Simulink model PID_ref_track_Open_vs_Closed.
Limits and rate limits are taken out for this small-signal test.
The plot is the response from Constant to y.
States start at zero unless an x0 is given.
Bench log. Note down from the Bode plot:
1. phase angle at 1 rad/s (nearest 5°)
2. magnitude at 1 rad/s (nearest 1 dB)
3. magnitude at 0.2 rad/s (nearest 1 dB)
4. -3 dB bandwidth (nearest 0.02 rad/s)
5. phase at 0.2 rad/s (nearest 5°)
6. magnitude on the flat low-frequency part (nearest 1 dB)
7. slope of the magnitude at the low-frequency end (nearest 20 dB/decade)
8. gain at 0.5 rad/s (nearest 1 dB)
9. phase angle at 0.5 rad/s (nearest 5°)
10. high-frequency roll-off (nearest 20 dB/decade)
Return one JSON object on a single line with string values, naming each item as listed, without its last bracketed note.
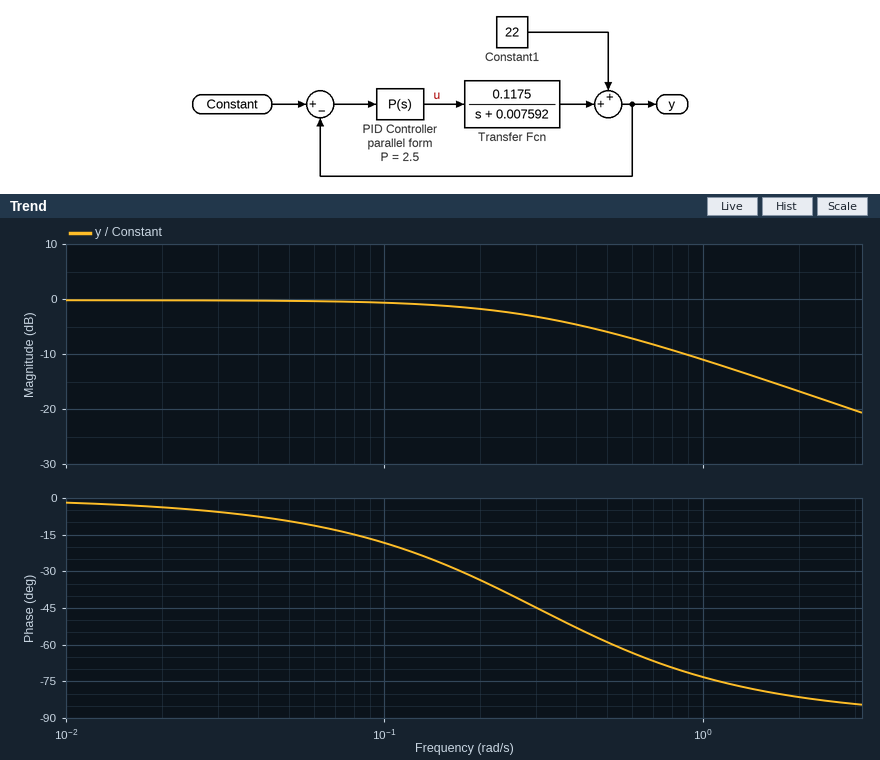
{"phase angle at 1 rad/s": "-75°", "magnitude at 1 rad/s": "-11 dB", "magnitude at 0.2 rad/s": "-2 dB", "-3 dB bandwidth": "0.30 rad/s", "phase at 0.2 rad/s": "-35°", "magnitude on the flat low-frequency part": "0 dB", "slope of the magnitude at the low-frequency end": "0 dB/decade", "gain at 0.5 rad/s": "-6 dB", "phase angle at 0.5 rad/s": "-60°", "high-frequency roll-off": "-20 dB/decade"}
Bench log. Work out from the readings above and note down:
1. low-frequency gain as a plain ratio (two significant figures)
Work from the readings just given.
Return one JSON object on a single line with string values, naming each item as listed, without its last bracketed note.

{"low-frequency gain as a plain ratio": "1.0"}
